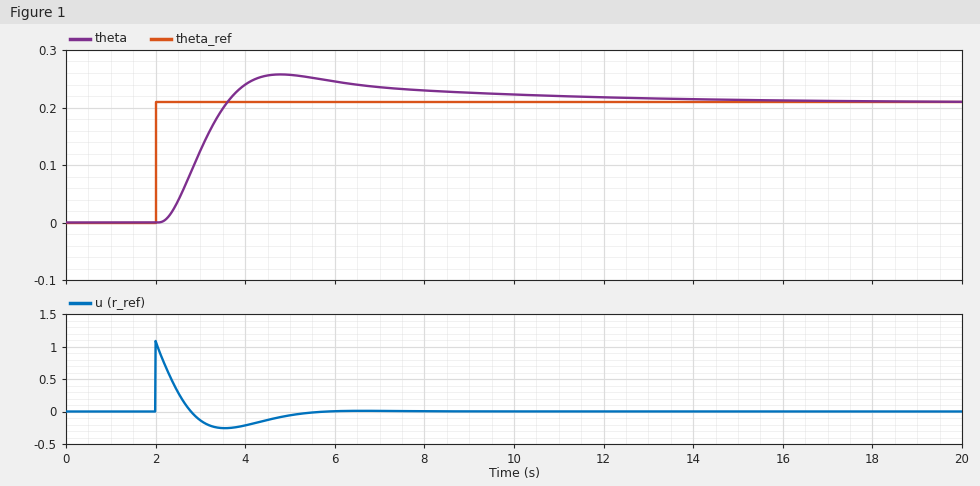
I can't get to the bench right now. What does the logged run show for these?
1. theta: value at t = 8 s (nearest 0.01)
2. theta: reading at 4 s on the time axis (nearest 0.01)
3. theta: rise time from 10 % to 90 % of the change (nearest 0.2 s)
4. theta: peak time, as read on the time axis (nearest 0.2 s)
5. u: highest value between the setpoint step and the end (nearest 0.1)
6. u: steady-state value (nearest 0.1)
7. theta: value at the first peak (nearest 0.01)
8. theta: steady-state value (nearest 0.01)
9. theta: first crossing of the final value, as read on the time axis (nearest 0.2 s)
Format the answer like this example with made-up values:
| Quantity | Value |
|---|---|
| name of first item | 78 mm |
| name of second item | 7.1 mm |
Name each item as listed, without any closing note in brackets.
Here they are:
| Quantity | Value |
|---|---|
| theta: value at t = 8 s | 0.23 |
| theta: reading at 4 s on the time axis | 0.24 |
| theta: rise time from 10 % to 90 % of the change | 1.0 s |
| theta: peak time, as read on the time axis | 4.8 s |
| u: highest value between the setpoint step and the end | 1.1 |
| u: steady-state value | 0.0 |
| theta: value at the first peak | 0.26 |
| theta: steady-state value | 0.21 |
| theta: first crossing of the final value, as read on the time axis | 3.6 s |
